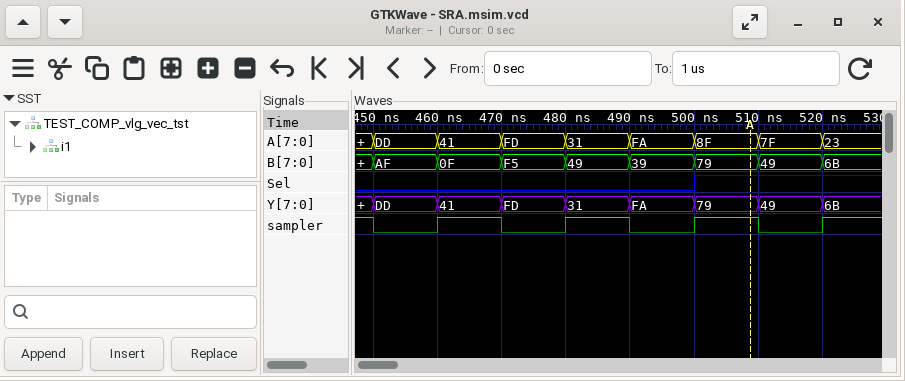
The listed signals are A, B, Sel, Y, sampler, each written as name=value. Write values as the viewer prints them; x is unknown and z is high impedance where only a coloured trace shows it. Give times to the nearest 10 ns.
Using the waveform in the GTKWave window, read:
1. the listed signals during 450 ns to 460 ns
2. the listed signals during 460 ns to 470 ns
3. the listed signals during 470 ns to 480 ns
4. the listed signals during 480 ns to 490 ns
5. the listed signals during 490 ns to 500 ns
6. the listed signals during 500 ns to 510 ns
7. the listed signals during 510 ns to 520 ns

A=DD, B=AF, Sel=0, Y=DD, sampler=0
A=41, B=0F, Sel=0, Y=41, sampler=1
A=FD, B=F5, Sel=0, Y=FD, sampler=0
A=31, B=49, Sel=0, Y=31, sampler=1
A=FA, B=39, Sel=0, Y=FA, sampler=0
A=8F, B=79, Sel=1, Y=79, sampler=1
A=7F, B=49, Sel=1, Y=49, sampler=0
